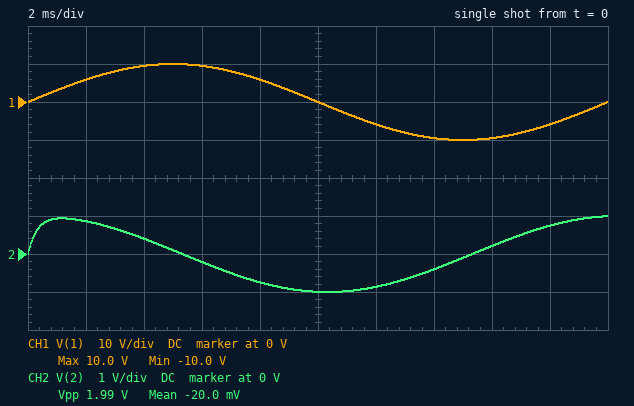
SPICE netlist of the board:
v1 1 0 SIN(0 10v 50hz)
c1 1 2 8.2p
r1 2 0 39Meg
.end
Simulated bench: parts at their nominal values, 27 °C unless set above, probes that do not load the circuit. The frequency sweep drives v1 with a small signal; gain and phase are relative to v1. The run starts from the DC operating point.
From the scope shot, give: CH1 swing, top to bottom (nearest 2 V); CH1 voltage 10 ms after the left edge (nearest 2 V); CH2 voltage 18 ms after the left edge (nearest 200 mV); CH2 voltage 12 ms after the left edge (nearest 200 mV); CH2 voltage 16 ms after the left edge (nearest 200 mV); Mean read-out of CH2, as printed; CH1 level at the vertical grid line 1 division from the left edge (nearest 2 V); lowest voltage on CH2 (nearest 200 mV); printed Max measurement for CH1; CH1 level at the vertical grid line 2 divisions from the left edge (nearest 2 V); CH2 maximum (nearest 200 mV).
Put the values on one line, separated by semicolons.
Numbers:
20 V; 0 V; 800 mV; -800 mV; 200 mV; -20.0 mV; 6 V; -1.0 V; 10.0 V; 10 V; 1.0 V
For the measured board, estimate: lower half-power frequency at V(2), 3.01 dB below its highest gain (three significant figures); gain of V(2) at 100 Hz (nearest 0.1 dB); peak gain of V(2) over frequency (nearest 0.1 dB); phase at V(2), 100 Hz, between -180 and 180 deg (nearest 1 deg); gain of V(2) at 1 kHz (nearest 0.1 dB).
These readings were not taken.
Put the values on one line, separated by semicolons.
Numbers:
498 Hz; -14.1 dB; 0 dB; 79 deg; -1.0 dB
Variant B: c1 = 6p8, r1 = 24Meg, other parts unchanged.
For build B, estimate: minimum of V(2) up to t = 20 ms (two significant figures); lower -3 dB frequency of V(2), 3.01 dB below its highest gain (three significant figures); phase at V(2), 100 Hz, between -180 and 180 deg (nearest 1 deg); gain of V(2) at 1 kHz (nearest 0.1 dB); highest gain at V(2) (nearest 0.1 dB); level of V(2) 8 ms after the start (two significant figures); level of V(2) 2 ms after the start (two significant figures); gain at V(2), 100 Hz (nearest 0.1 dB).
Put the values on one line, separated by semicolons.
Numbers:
-510 mV; 975 Hz; 84 deg; -2.9 dB; 0 dB; -400 mV; 430 mV; -19.8 dB
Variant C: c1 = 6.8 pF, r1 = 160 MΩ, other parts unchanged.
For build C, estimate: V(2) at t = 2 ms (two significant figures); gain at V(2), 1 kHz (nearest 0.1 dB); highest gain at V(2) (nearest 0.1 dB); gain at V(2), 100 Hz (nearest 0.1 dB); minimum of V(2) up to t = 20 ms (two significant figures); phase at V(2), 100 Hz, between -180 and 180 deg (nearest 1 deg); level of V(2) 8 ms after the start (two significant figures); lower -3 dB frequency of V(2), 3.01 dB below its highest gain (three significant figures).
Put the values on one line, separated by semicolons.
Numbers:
2.6 V; -0.1 dB; 0 dB; -5.0 dB; -3.2 V; 56 deg; -1.9 V; 146 Hz
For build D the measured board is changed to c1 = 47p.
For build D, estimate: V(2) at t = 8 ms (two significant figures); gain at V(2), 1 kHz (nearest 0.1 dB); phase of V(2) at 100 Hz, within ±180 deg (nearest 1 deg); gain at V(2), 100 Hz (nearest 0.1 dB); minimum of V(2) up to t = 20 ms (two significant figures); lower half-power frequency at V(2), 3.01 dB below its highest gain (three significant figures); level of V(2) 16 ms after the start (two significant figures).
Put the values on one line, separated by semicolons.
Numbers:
-2.1 V; 0 dB; 41 deg; -2.4 dB; -5.0 V; 86.8 Hz; -1.0 V
